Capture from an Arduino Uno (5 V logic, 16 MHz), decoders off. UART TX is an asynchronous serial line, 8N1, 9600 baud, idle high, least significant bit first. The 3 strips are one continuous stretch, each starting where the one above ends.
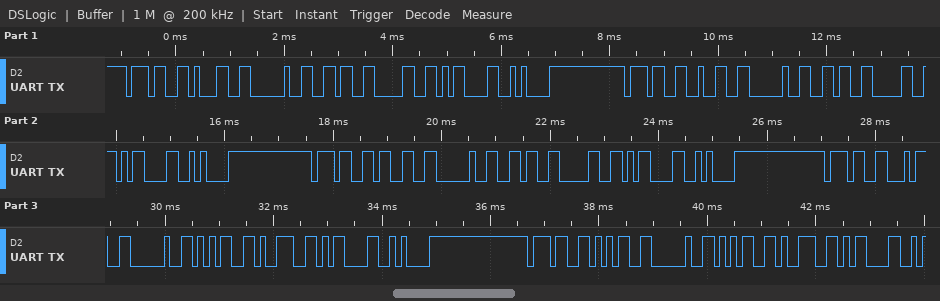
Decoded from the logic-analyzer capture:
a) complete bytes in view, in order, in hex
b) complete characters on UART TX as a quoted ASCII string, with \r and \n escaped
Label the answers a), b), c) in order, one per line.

a) 37 31 20 36 30 0D 0A 37 32 20 36 30 0D 0A 37 33 20 36 30 0D 0A 37 34 20 35 39 0D 0A 37 35 20 35 39 0D
b) "71 60\r\n72 60\r\n73 60\r\n74 59\r\n75 59\r"
